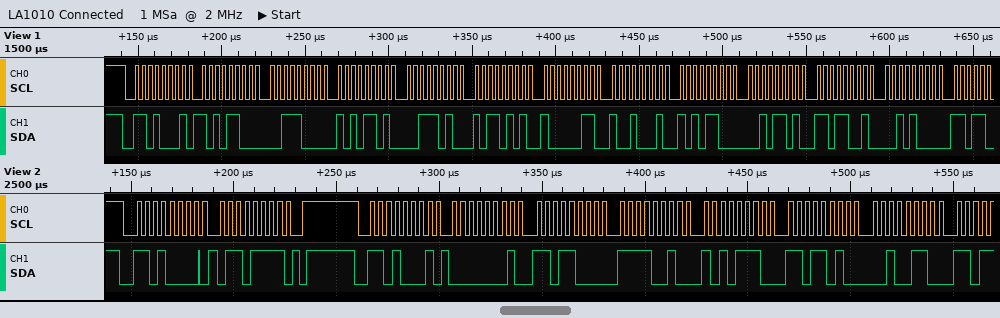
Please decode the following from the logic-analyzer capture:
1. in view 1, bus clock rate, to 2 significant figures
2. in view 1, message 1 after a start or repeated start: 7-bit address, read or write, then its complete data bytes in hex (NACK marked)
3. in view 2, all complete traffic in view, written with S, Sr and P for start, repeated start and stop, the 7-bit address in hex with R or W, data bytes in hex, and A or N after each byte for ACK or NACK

250 kHz
0x68 read: AC 38 AD 3A B5 83 91 AC 2D D9 28
S 68W A 6F A P S 68R A 01 A D8 A F2 A AE A DA A 26 A
